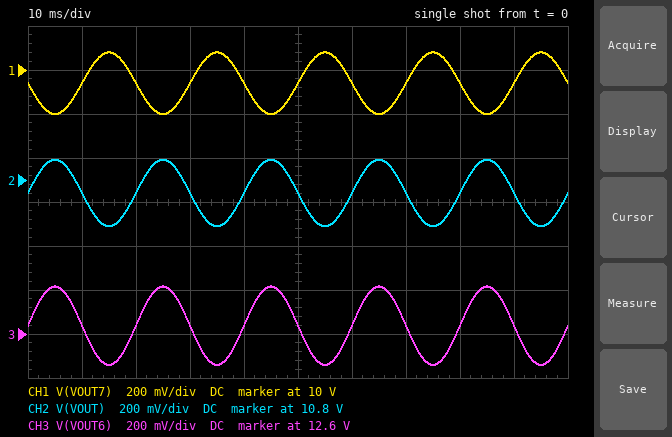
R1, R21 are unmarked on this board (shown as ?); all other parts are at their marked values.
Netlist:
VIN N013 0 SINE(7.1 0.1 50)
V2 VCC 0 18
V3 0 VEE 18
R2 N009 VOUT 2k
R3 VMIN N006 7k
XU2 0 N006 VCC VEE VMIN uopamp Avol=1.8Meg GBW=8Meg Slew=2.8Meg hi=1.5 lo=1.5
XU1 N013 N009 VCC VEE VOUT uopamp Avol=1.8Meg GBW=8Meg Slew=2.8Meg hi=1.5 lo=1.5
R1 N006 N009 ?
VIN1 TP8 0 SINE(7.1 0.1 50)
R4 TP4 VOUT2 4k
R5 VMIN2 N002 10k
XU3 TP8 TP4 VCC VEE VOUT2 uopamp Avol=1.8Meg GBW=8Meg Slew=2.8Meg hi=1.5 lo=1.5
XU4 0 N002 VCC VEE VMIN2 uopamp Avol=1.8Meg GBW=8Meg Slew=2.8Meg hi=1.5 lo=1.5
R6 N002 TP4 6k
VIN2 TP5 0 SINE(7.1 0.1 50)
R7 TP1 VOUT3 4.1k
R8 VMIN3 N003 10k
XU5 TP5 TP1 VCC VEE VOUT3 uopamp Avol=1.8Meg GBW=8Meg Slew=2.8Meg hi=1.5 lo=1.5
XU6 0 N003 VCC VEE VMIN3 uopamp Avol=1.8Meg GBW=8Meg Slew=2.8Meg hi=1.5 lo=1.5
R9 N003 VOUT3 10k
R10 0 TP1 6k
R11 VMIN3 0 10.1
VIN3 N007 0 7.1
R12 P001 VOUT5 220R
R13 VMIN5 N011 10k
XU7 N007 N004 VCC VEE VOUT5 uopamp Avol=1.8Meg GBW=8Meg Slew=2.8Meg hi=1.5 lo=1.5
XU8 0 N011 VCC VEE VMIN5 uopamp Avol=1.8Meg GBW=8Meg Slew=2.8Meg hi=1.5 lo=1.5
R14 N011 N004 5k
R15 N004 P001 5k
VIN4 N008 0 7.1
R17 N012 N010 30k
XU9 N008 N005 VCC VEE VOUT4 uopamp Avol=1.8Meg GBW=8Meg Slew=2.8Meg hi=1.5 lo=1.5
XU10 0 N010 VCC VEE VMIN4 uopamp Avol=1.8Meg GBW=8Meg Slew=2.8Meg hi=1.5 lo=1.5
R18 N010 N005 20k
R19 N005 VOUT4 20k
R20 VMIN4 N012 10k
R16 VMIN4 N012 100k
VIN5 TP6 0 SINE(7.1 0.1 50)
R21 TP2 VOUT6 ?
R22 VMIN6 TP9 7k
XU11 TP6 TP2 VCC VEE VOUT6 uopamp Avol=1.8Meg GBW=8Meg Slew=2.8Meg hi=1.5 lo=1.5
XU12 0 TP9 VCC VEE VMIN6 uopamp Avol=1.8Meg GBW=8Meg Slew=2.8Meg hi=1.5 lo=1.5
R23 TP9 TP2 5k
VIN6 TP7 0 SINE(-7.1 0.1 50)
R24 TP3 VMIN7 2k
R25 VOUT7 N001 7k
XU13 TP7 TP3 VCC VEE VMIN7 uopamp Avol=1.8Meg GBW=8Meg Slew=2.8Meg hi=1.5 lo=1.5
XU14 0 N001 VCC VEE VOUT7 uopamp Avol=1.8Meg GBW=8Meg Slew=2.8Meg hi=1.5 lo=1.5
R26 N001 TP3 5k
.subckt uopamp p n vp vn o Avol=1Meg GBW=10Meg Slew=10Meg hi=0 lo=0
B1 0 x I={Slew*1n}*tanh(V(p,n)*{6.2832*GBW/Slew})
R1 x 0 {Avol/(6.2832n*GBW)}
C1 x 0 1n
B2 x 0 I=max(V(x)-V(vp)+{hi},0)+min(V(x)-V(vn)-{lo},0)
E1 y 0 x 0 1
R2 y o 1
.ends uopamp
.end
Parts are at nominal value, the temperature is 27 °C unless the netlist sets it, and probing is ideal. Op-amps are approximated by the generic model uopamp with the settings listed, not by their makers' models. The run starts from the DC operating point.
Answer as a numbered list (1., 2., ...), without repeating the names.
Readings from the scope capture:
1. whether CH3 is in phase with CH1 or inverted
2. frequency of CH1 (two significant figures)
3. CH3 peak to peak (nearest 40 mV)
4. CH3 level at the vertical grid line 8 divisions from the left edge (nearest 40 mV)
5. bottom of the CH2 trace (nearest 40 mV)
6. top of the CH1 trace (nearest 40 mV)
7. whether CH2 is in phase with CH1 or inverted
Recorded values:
1. inverted
2. 50 Hz
3. 360 mV
4. 12.64 V
5. 10.60 V
6. 10.08 V
7. inverted
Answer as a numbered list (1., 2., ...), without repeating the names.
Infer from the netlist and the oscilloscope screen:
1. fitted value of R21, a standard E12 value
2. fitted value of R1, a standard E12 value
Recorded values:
1. 3.9 kΩ
2. 3.9 kΩ
